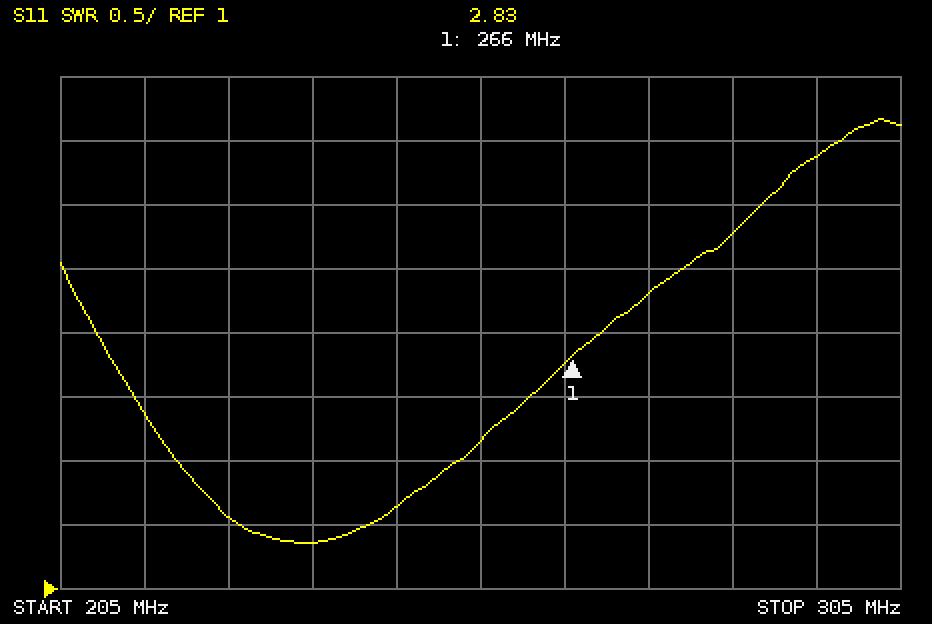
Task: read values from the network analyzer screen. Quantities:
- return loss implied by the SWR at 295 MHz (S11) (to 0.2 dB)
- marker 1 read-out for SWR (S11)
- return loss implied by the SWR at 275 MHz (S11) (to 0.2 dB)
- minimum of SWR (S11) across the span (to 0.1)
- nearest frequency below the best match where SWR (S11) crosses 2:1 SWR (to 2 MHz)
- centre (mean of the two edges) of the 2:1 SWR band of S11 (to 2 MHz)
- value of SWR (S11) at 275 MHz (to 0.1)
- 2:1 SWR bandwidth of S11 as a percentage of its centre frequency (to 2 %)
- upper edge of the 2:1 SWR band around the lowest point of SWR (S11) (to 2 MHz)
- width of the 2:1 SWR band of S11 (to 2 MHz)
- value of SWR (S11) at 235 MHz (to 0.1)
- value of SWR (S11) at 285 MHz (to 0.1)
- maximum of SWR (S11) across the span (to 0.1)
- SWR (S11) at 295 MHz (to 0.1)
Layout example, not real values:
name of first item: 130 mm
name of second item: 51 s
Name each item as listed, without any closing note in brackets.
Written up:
return loss implied by the SWR at 295 MHz (S11): 4.0 dB
marker 1 read-out for SWR: 2.83
return loss implied by the SWR at 275 MHz (S11): 5.4 dB
minimum of SWR (S11) across the span: 1.4
nearest frequency below the best match where SWR (S11) crosses 2:1 SWR: 218 MHz
centre (mean of the two edges) of the 2:1 SWR band of S11: 236 MHz
value of SWR (S11) at 275 MHz: 3.3
2:1 SWR bandwidth of S11 as a percentage of its centre frequency: 14 %
upper edge of the 2:1 SWR band around the lowest point of SWR (S11): 252 MHz
width of the 2:1 SWR band of S11: 34 MHz
value of SWR (S11) at 235 MHz: 1.4
value of SWR (S11) at 285 MHz: 3.8
maximum of SWR (S11) across the span: 4.7
SWR (S11) at 295 MHz: 4.4
